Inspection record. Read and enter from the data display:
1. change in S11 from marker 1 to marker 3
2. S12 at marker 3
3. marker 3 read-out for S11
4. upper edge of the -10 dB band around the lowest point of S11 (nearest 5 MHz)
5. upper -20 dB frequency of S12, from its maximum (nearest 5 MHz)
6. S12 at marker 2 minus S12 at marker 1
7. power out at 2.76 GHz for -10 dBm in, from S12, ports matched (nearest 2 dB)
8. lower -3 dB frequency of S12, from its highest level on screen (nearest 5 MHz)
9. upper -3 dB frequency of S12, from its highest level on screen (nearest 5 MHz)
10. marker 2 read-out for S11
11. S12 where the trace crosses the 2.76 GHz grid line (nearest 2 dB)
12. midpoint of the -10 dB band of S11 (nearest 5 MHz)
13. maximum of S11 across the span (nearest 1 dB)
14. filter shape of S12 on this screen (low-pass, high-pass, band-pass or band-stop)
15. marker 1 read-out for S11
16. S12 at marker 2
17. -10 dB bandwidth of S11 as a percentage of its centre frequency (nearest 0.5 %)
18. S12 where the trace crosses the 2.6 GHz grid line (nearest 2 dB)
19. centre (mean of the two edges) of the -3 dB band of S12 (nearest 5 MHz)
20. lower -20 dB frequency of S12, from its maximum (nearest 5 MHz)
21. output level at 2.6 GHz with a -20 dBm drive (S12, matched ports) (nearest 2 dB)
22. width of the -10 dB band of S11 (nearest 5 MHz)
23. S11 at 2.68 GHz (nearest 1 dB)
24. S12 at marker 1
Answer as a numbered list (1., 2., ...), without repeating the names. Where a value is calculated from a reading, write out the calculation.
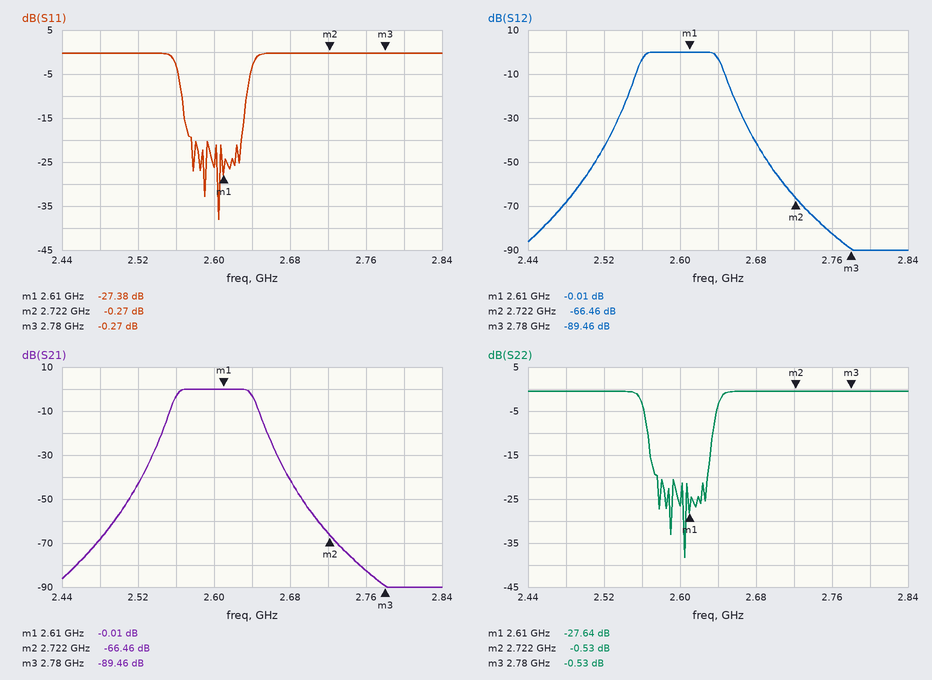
1. -0.27 − (-27.38) = 27.11 dB
2. -89.46 dB
3. -0.27 dB
4. 2.635 GHz
5. 2.655 GHz
6. -66.46 − (-0.01) = -66.45 dB
7. -10 dBm + (-82 dB) = -92 dBm
8. 2.560 GHz
9. 2.640 GHz
10. -0.27 dB
11. -82 dB
12. 2.600 GHz
13. 0 dB
14. band-pass
15. -27.38 dB
16. -66.46 dB
17. 70 MHz / 2.6 GHz ≈ 2.69 %, so 2.5 % to the nearest 0.5 %
18. 0 dB
19. 2.600 GHz
20. 2.545 GHz
21. -20 dBm + (0 dB) = -20 dBm
22. 2.635 GHz − 2.565 GHz = 70 MHz
23. 0 dB
24. -0.01 dB
